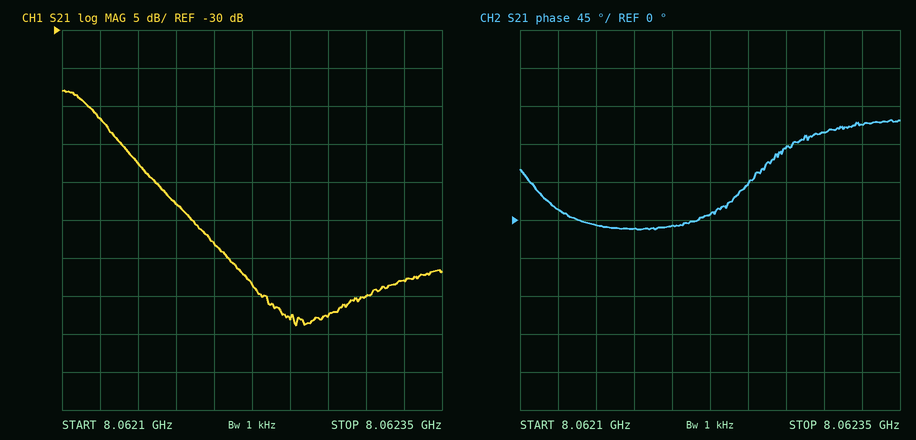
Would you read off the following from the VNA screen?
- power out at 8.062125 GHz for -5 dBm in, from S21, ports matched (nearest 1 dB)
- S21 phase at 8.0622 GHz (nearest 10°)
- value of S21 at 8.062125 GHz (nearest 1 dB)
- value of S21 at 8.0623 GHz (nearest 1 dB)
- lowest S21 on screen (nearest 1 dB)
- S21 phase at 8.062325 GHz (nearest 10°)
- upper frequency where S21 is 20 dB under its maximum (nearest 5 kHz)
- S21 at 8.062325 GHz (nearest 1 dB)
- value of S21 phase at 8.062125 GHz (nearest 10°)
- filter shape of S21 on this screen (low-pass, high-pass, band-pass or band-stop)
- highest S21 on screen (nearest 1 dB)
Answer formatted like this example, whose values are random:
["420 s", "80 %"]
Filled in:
["-47 dBm", "-10°", "-42 dB", "-65 dB", "-69 dB", "110°", "8.062200 GHz", "-63 dB", "10°", "low-pass", "-38 dB"]
